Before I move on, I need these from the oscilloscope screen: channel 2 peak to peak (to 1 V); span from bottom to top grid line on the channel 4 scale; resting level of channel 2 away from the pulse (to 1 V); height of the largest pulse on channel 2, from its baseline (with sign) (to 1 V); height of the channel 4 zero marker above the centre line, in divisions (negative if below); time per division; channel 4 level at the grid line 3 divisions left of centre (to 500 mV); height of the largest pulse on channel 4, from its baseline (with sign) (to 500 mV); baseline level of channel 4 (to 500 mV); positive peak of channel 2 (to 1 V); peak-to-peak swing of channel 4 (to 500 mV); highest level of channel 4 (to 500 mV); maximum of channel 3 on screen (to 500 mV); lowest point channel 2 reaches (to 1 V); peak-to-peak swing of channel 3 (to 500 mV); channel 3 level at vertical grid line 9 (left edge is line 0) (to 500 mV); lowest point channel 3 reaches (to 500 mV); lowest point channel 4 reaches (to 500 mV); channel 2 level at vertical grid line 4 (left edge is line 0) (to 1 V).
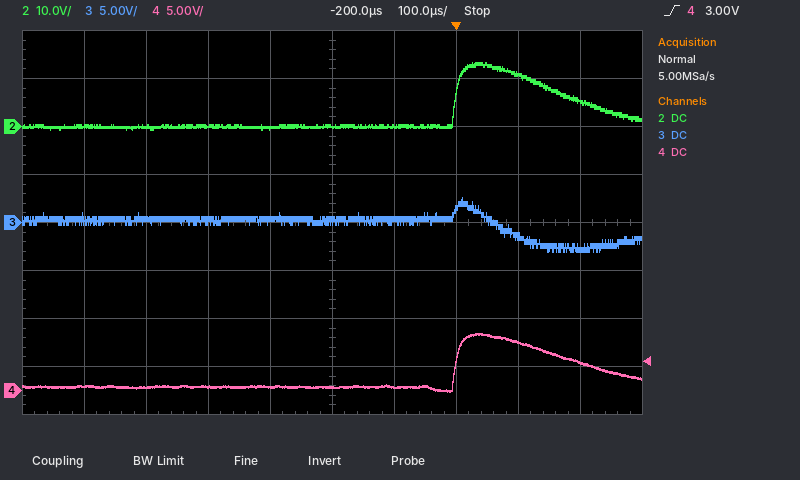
14 V
40 V
0 V
+13 V
-3.5 div
100 µs
500 mV
+5.5 V
500 mV
13 V
6.0 V
6.0 V
2.5 V
-1 V
5.5 V
-2.5 V
-3.0 V
0.0 V
0 V
